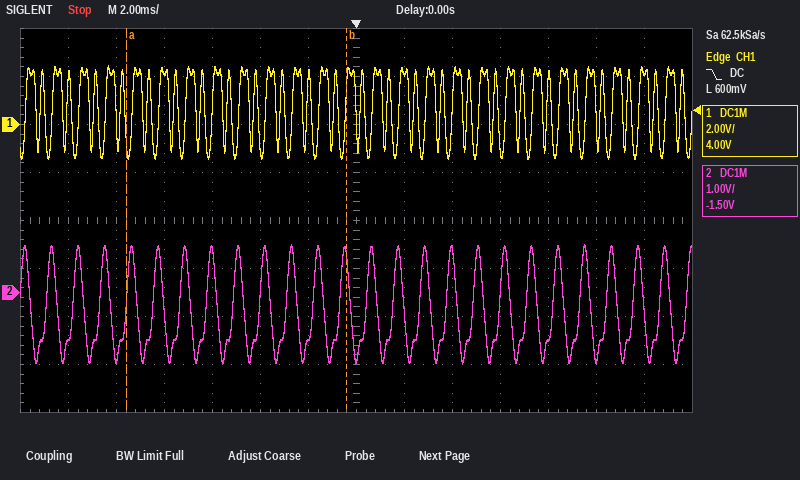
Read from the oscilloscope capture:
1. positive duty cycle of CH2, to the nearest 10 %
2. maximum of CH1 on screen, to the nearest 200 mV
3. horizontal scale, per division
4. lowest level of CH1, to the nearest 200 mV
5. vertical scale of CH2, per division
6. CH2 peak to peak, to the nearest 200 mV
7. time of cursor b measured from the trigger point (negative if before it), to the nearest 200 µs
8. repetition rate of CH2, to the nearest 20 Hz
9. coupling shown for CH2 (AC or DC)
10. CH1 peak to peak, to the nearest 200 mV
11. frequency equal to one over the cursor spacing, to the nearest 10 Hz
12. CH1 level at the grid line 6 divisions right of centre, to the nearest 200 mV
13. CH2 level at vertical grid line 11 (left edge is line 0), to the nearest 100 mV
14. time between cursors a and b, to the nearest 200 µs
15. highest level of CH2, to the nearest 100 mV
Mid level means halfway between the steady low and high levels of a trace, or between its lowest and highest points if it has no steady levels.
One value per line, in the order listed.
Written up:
40 %
2.4 V
2 ms
-1.4 V
1 V
2.4 V
-400 µs
900 Hz
DC
3.8 V
110 Hz
2.2 V
-1.0 V
9.2 ms
1.0 V
